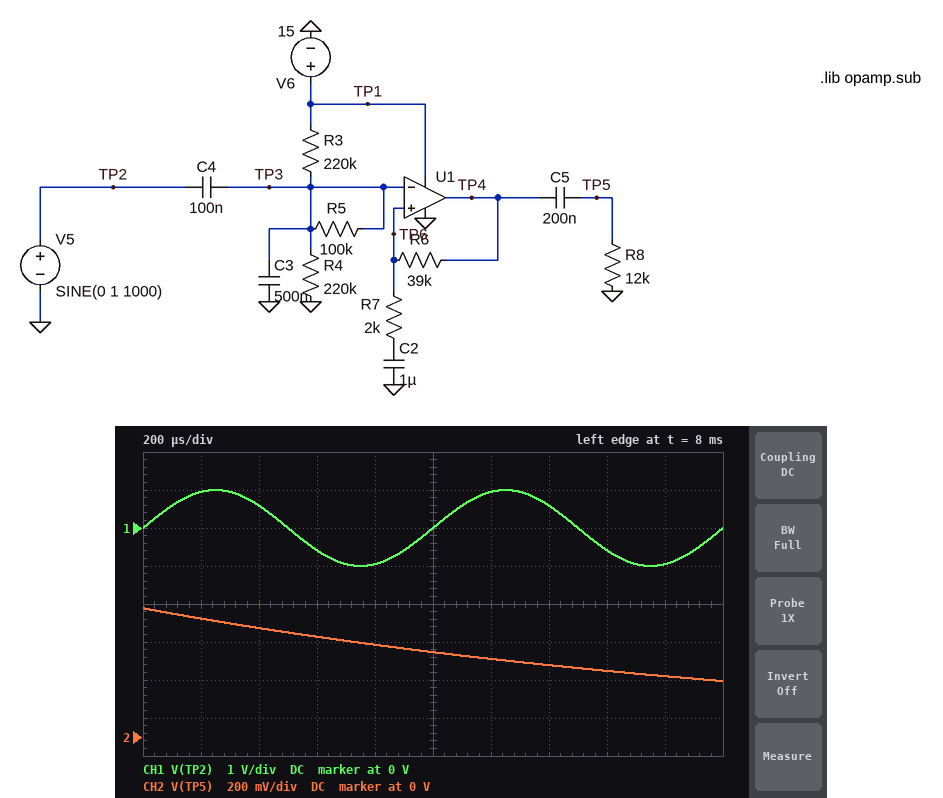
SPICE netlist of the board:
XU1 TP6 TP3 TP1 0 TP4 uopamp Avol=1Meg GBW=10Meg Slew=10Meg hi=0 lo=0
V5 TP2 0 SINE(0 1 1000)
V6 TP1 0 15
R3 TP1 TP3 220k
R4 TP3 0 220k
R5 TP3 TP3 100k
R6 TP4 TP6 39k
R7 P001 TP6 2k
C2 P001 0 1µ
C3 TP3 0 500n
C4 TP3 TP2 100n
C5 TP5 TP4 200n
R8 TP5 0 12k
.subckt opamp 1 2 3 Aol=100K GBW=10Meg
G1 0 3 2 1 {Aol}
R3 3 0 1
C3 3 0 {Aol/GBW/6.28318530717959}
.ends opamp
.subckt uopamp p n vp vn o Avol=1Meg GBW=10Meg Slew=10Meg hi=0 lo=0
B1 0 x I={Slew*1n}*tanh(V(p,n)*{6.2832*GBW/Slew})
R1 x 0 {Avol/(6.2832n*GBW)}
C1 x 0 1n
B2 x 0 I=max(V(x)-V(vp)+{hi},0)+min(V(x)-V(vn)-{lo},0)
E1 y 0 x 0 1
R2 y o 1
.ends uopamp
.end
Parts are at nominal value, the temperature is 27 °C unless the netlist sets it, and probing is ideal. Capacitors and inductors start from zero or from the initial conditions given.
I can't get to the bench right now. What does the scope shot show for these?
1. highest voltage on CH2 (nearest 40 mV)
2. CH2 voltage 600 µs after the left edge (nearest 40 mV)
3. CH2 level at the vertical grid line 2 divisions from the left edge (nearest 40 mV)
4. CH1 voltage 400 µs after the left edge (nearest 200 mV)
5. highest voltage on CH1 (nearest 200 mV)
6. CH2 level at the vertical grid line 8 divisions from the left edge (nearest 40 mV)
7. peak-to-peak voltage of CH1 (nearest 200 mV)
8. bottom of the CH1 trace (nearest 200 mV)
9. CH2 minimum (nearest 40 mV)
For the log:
680 mV
520 mV
560 mV
600 mV
1.0 V
360 mV
2.0 V
-1.0 V
280 mV
